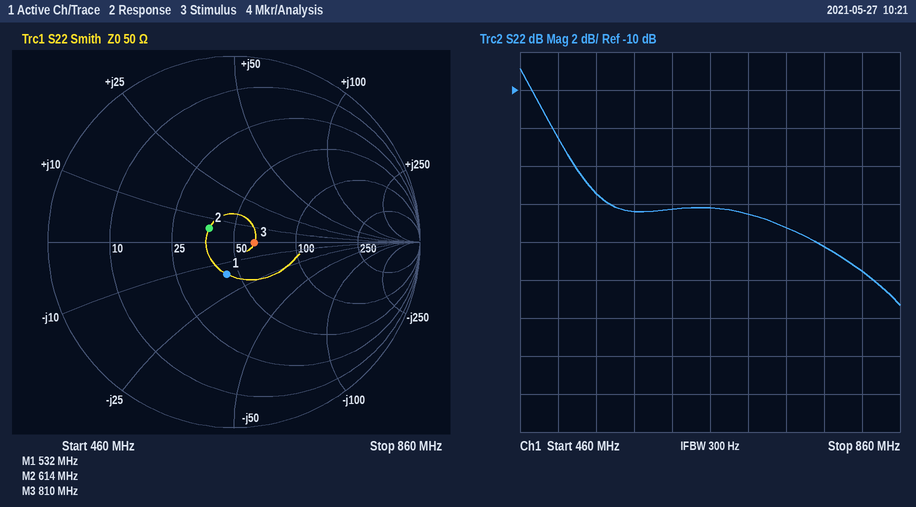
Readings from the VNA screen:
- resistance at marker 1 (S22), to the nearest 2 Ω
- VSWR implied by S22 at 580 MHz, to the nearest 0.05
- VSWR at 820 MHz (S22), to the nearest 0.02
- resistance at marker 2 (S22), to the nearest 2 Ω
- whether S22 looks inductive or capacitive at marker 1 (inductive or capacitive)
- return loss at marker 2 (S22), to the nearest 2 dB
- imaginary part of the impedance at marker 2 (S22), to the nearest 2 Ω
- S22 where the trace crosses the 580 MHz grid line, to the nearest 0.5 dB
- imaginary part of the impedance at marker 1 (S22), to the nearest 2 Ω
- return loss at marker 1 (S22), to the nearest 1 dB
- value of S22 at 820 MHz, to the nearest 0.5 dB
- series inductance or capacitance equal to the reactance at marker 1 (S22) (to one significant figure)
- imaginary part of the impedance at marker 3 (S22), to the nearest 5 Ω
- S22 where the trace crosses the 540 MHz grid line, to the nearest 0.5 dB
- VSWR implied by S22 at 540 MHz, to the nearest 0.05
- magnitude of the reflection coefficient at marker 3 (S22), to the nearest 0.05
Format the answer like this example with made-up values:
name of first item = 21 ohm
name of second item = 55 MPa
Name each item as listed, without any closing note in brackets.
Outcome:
resistance at marker 1 (S22), to the nearest 2 Ω = 44 Ω
VSWR implied by S22 at 580 MHz, to the nearest 0.05 = 1.35
VSWR at 820 MHz (S22), to the nearest 0.02 = 1.24
resistance at marker 2 (S22), to the nearest 2 Ω = 38 Ω
whether S22 looks inductive or capacitive at marker 1 = capacitive
return loss at marker 2 (S22), to the nearest 2 dB = 16 dB
imaginary part of the impedance at marker 2 (S22), to the nearest 2 Ω = +6 Ω
S22 where the trace crosses the 580 MHz grid line, to the nearest 0.5 dB = -16.5 dB
imaginary part of the impedance at marker 1 (S22), to the nearest 2 Ω = -16 Ω
return loss at marker 1 (S22), to the nearest 1 dB = 15 dB
value of S22 at 820 MHz, to the nearest 0.5 dB = -19.5 dB
series inductance or capacitance equal to the reactance at marker 1 (S22) = 20 pF
imaginary part of the impedance at marker 3 (S22), to the nearest 5 Ω = 0 Ω
S22 where the trace crosses the 540 MHz grid line, to the nearest 0.5 dB = -15.5 dB
VSWR implied by S22 at 540 MHz, to the nearest 0.05 = 1.40
magnitude of the reflection coefficient at marker 3 (S22), to the nearest 0.05 = 0.10
